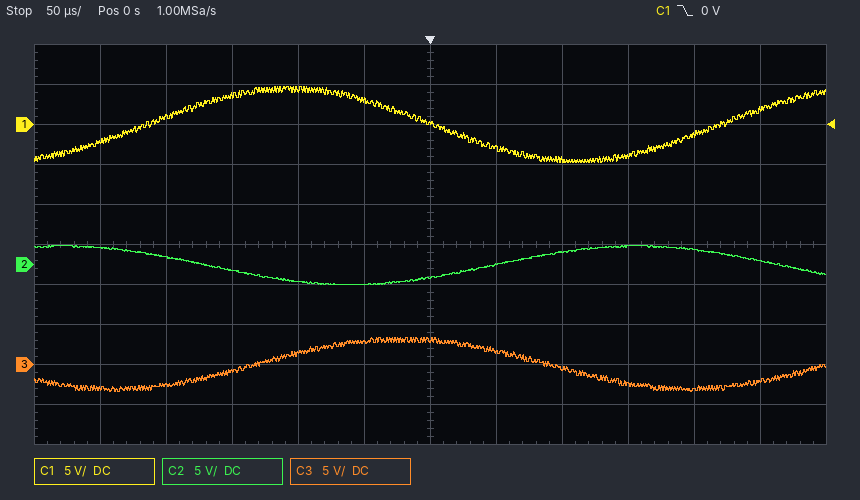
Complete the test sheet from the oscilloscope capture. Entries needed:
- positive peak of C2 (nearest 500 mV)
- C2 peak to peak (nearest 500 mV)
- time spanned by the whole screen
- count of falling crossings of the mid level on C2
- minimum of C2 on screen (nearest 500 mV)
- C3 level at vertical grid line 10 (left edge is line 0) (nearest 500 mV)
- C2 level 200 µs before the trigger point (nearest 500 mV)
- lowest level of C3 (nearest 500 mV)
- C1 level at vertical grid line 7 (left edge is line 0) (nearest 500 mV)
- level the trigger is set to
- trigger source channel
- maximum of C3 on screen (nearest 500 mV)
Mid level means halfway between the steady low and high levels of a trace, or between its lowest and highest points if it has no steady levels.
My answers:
2.5 V
5.0 V
600 µs
2
-2.5 V
-3.0 V
1.0 V
-3.5 V
-3.0 V
0 V
C1
3.5 V
